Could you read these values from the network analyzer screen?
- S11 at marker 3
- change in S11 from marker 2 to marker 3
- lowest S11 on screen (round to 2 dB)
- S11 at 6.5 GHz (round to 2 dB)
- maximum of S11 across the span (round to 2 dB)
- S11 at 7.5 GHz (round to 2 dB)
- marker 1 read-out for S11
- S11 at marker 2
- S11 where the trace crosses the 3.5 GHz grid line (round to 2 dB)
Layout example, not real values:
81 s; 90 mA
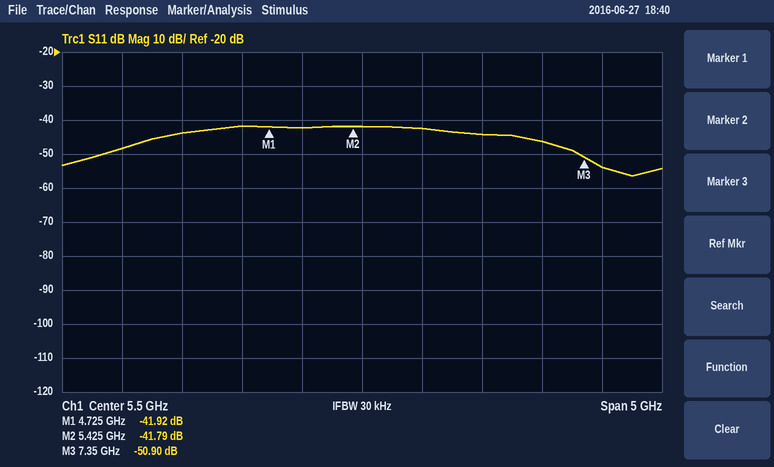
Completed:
-50.90 dB; -9.11 dB; -56 dB; -44 dB; -42 dB; -54 dB; -41.92 dB; -41.79 dB; -48 dB
